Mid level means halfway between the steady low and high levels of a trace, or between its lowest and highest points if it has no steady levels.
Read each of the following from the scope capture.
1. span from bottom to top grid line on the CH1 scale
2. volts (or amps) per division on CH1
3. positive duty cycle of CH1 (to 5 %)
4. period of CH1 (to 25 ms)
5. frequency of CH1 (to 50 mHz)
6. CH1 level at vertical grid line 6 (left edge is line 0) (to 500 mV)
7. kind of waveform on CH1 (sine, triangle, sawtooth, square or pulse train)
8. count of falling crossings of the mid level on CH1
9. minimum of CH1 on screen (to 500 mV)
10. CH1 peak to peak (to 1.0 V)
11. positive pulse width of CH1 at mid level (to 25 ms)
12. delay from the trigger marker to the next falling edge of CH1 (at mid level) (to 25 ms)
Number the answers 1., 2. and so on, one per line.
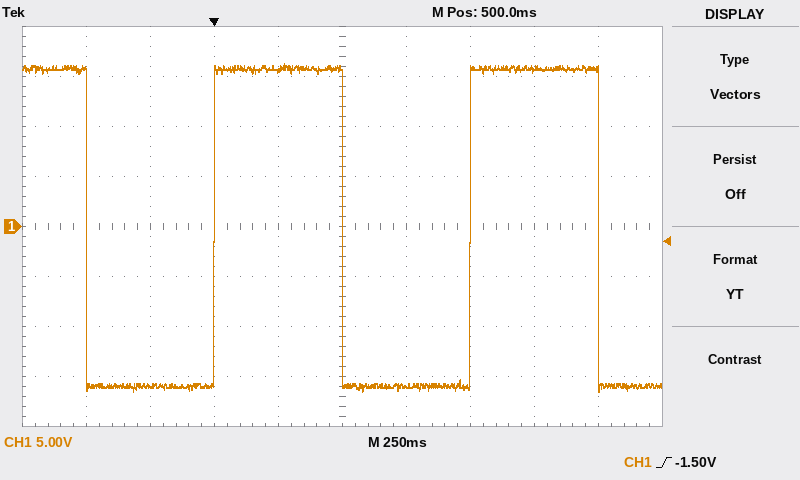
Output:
1. 40 V
2. 5 V
3. 50 %
4. 1.000 s
5. 1.00 Hz
6. -16.0 V
7. square
8. 3
9. -16.5 V
10. 33.0 V
11. 500 ms
12. 500 ms
